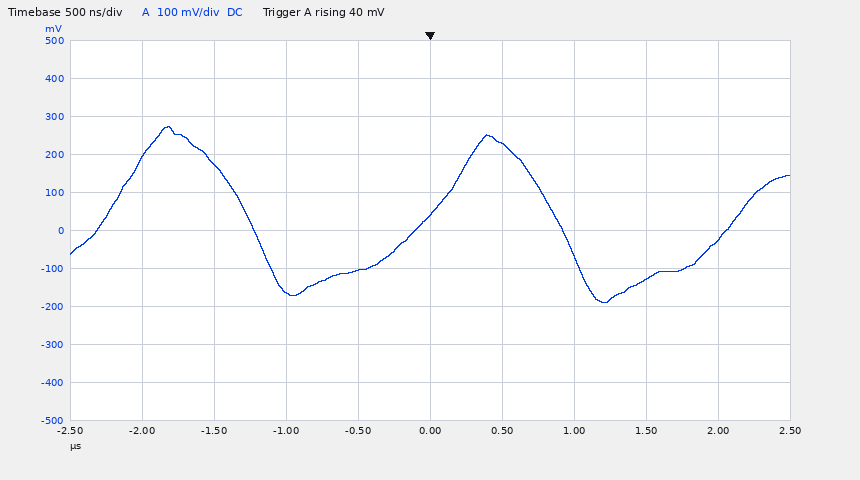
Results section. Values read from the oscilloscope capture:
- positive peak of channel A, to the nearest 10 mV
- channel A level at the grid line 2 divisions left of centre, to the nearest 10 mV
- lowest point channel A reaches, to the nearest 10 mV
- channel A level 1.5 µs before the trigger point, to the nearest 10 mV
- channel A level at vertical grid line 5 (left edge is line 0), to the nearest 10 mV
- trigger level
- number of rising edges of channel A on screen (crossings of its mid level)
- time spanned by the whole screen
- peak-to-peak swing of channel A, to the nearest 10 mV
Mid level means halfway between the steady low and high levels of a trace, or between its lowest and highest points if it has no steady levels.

270 mV
-160 mV
-190 mV
170 mV
40 mV
40 mV
3
5 µs
460 mV
